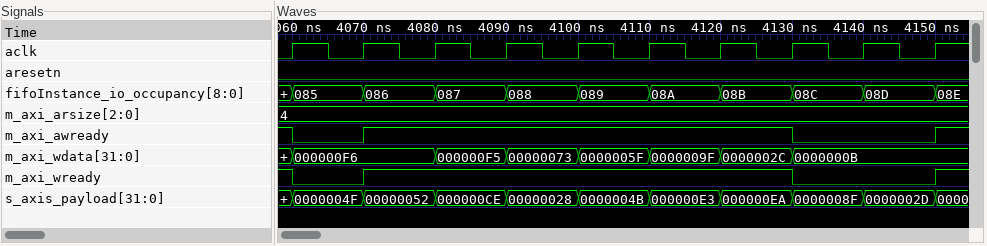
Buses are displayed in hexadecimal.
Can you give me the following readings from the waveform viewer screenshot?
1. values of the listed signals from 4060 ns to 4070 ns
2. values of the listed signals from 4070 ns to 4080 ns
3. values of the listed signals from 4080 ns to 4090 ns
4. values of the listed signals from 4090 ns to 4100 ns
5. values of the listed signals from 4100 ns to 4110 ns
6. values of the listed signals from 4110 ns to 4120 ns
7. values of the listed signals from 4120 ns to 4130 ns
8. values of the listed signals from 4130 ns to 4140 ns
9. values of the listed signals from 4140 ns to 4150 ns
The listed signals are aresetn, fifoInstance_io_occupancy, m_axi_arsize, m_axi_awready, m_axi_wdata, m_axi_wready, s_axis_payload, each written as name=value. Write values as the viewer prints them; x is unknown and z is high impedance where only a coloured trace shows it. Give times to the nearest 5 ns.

aresetn=0, fifoInstance_io_occupancy=085, m_axi_arsize=4, m_axi_awready=0, m_axi_wdata=000000F6, m_axi_wready=0, s_axis_payload=0000004F
aresetn=0, fifoInstance_io_occupancy=086, m_axi_arsize=4, m_axi_awready=1, m_axi_wdata=000000F6, m_axi_wready=1, s_axis_payload=00000052
aresetn=0, fifoInstance_io_occupancy=087, m_axi_arsize=4, m_axi_awready=1, m_axi_wdata=000000F5, m_axi_wready=1, s_axis_payload=000000CE
aresetn=0, fifoInstance_io_occupancy=088, m_axi_arsize=4, m_axi_awready=1, m_axi_wdata=00000073, m_axi_wready=1, s_axis_payload=00000028
aresetn=0, fifoInstance_io_occupancy=089, m_axi_arsize=4, m_axi_awready=1, m_axi_wdata=0000005F, m_axi_wready=1, s_axis_payload=0000004B
aresetn=0, fifoInstance_io_occupancy=08A, m_axi_arsize=4, m_axi_awready=1, m_axi_wdata=0000009F, m_axi_wready=1, s_axis_payload=000000E3
aresetn=0, fifoInstance_io_occupancy=08B, m_axi_arsize=4, m_axi_awready=1, m_axi_wdata=0000002C, m_axi_wready=1, s_axis_payload=000000EA
aresetn=0, fifoInstance_io_occupancy=08C, m_axi_arsize=4, m_axi_awready=0, m_axi_wdata=0000000B, m_axi_wready=0, s_axis_payload=0000008F
aresetn=0, fifoInstance_io_occupancy=08D, m_axi_arsize=4, m_axi_awready=0, m_axi_wdata=0000000B, m_axi_wready=0, s_axis_payload=0000002D
